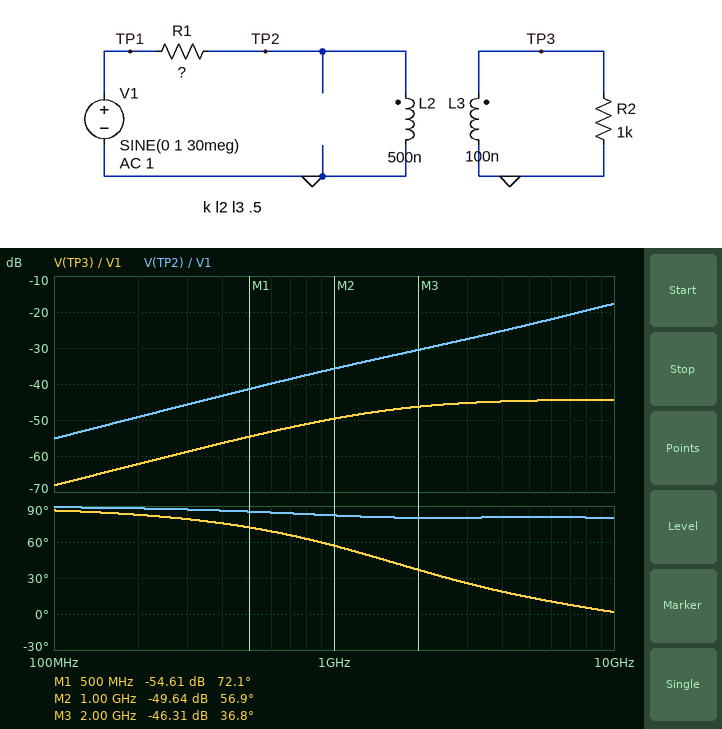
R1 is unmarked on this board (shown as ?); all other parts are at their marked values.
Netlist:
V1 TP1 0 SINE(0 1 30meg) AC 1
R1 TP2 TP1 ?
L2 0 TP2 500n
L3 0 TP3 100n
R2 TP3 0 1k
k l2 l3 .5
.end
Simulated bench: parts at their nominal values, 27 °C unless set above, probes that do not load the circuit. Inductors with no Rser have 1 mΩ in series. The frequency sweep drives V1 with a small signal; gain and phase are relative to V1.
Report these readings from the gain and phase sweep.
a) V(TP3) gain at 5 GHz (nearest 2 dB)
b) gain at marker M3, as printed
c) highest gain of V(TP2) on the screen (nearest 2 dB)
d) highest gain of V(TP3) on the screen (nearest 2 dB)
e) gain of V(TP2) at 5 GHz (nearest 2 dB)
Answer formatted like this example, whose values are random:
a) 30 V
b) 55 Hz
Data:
a) -44 dB
b) -46.31 dB
c) -18 dB
d) -44 dB
e) -24 dB
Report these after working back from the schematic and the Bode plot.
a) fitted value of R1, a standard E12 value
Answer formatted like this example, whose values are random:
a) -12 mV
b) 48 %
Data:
a) 180 kΩ
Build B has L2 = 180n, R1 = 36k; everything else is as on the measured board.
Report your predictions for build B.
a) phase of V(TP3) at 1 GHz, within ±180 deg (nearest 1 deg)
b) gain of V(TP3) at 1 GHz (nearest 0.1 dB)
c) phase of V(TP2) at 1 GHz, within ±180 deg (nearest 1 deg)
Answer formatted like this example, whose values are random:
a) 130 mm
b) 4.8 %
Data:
a) 56 deg
b) -40.1 dB
c) 81 deg
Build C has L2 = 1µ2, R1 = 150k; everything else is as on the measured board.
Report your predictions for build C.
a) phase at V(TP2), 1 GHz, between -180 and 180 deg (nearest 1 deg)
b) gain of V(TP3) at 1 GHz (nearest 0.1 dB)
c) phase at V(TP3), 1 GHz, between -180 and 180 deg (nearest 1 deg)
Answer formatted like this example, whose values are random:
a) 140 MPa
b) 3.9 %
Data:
a) 80 deg
b) -44.3 dB
c) 55 deg
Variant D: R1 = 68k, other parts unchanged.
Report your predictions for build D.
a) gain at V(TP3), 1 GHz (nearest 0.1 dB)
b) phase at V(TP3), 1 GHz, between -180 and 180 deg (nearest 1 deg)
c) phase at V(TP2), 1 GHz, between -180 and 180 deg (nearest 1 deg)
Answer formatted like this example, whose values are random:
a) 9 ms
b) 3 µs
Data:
a) -41.2 dB
b) 55 deg
c) 81 deg
